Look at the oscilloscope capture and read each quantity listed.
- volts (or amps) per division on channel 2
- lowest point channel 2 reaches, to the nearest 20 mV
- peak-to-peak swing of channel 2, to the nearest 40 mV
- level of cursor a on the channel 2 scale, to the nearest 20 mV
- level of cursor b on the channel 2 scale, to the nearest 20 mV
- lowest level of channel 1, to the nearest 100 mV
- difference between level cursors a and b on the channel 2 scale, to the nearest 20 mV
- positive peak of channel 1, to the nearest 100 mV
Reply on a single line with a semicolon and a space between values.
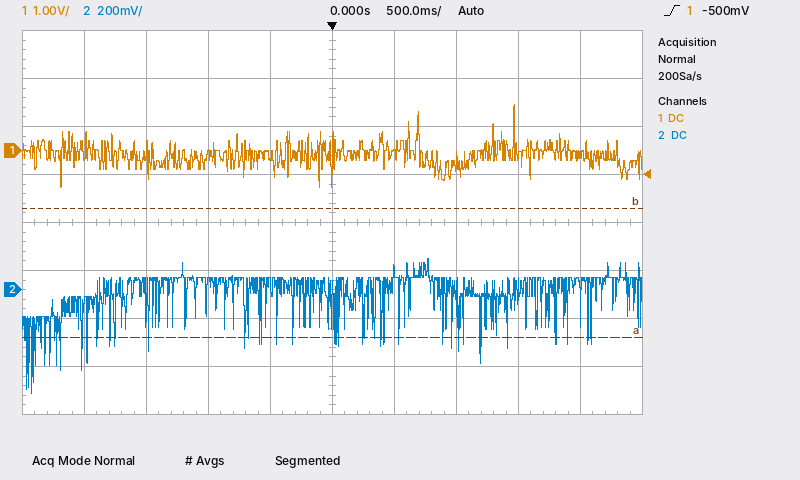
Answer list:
200 mV; -440 mV; 560 mV; -200 mV; 340 mV; -800 mV; 540 mV; 1.0 V
